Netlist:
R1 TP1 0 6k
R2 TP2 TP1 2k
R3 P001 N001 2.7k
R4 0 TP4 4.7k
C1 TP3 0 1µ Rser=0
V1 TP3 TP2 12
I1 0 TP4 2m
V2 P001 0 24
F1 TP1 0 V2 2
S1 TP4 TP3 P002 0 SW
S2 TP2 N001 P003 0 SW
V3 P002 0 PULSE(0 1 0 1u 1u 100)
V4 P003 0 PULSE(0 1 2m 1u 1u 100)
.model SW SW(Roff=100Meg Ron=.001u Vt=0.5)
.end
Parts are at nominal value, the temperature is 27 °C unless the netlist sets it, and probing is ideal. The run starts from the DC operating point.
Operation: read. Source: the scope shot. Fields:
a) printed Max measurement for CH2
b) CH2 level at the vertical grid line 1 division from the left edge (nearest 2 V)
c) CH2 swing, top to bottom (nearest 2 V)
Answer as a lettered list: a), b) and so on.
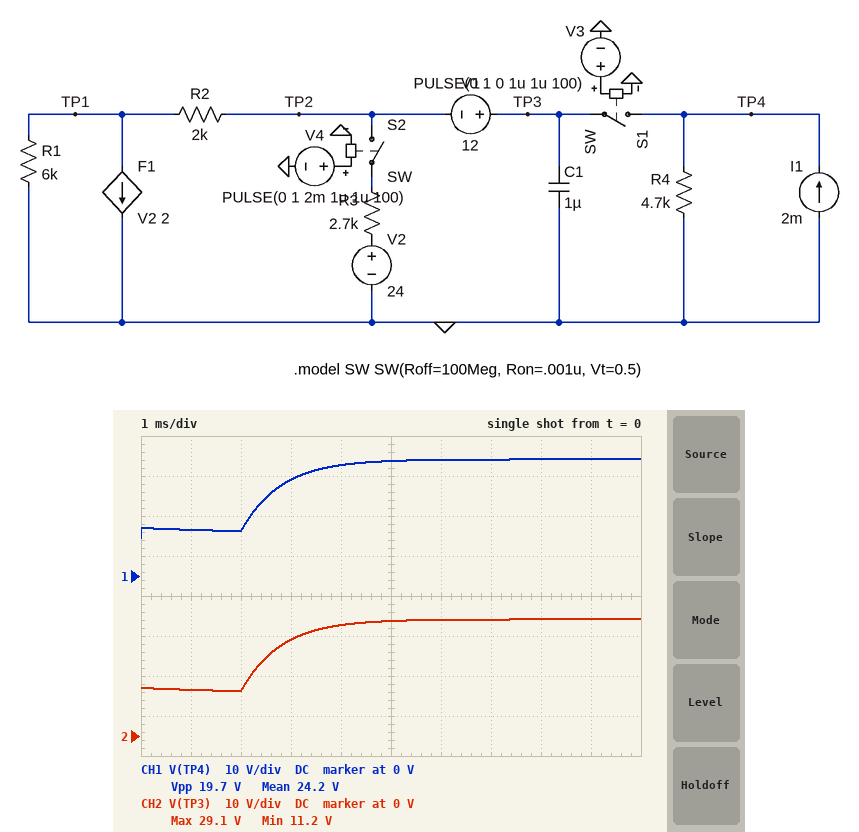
a) 29.1 V
b) 12 V
c) 18 V
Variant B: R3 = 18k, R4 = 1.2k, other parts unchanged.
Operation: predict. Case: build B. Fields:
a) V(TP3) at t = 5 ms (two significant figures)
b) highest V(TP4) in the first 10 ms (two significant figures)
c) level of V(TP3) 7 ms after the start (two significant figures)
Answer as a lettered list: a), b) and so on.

a) 7.6 V
b) 12 V
c) 7.7 V
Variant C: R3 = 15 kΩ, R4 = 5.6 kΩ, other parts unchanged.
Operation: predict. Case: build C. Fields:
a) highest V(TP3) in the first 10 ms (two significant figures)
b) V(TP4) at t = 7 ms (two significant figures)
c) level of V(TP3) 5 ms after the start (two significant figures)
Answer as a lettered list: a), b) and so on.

a) 20 V
b) 19 V
c) 18 V
